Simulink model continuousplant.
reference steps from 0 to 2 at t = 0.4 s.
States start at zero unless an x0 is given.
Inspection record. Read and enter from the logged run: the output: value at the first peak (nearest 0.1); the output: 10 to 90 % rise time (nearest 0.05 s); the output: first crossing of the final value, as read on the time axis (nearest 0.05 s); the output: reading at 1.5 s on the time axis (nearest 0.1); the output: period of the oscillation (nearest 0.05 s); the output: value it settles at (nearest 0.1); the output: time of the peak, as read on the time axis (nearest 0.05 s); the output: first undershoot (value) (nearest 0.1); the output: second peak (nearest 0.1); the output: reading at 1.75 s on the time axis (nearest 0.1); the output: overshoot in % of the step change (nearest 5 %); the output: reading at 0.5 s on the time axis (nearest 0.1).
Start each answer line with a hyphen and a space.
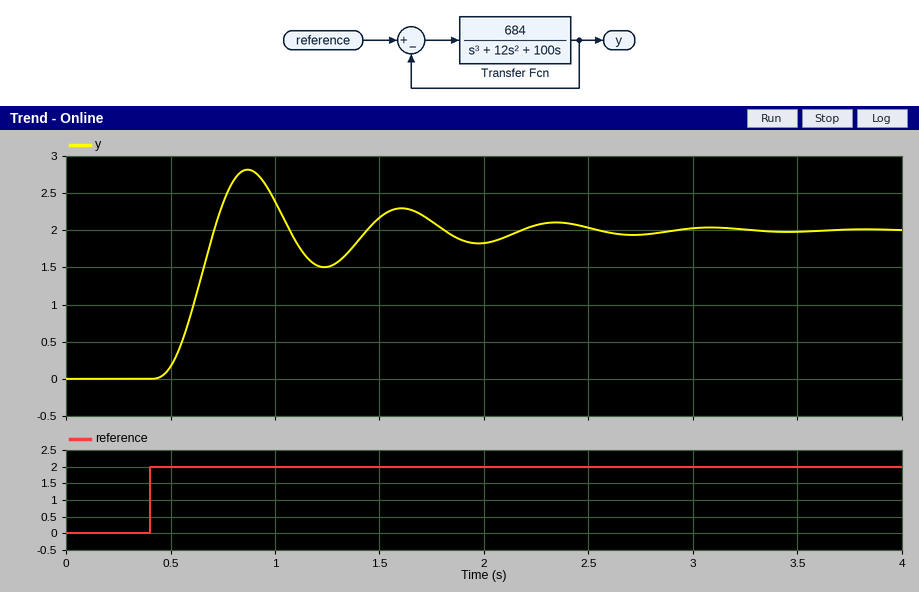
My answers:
- 2.8
- 0.20 s
- 0.70 s
- 2.2
- 0.75 s
- 2.0
- 0.85 s
- 1.5
- 2.3
- 2.1
- 40 %
- 0.2
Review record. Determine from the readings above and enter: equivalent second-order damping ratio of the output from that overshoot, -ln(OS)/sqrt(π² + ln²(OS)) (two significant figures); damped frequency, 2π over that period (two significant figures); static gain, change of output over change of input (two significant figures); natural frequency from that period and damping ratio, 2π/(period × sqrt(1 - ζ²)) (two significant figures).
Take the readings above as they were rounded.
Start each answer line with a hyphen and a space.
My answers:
- 0.28
- 8.4 rad/s
- 1.0
- 8.7 rad/s
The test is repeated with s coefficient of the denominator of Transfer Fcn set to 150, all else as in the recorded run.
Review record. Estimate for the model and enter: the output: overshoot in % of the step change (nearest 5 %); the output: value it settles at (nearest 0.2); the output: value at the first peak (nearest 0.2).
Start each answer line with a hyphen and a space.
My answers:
- 10 %
- 2.0
- 2.2
